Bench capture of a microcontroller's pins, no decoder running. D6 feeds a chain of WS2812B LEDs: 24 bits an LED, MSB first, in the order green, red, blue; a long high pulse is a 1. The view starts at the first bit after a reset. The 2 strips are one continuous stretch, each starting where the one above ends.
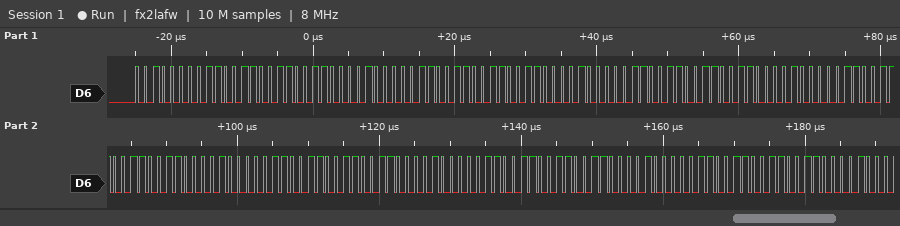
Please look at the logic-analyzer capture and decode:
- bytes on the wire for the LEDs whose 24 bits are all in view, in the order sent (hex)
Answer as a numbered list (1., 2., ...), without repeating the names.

1. 20 CC CC 20 CC CC 20 CC CC 20 CC CC 20 CC CC 20 CC CC 20 CC CC
